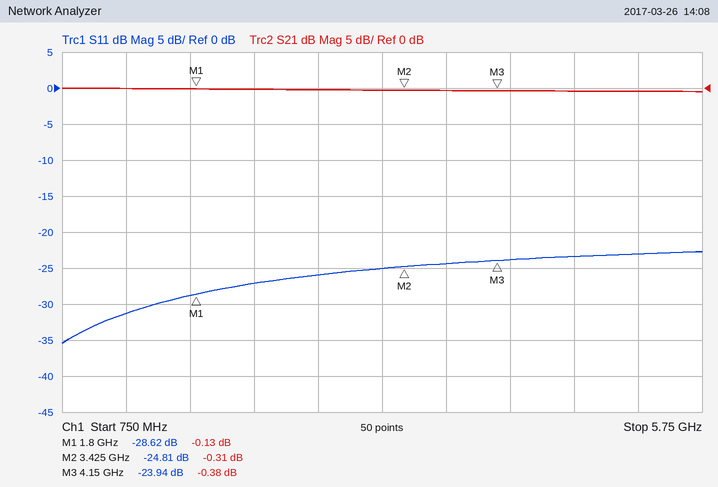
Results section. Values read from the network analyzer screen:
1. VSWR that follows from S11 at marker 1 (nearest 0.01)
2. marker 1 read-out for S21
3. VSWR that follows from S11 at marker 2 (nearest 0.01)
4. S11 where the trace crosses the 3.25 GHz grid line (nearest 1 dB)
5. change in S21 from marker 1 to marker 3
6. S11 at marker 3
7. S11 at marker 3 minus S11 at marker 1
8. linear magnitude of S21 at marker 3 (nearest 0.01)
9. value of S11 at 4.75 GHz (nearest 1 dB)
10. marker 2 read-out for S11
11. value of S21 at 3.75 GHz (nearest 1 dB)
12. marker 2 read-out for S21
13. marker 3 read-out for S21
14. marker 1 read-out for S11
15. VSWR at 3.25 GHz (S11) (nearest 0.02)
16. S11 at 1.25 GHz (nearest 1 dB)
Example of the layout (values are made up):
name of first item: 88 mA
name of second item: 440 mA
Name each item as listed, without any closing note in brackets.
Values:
VSWR that follows from S11 at marker 1: 1.08
marker 1 read-out for S21: -0.13 dB
VSWR that follows from S11 at marker 2: 1.12
S11 where the trace crosses the 3.25 GHz grid line: -25 dB
change in S21 from marker 1 to marker 3: -0.25 dB
S11 at marker 3: -23.94 dB
S11 at marker 3 minus S11 at marker 1: 4.68 dB
linear magnitude of S21 at marker 3: 0.96
value of S11 at 4.75 GHz: -23 dB
marker 2 read-out for S11: -24.81 dB
value of S21 at 3.75 GHz: 0 dB
marker 2 read-out for S21: -0.31 dB
marker 3 read-out for S21: -0.38 dB
marker 1 read-out for S11: -28.62 dB
VSWR at 3.25 GHz (S11): 1.12
S11 at 1.25 GHz: -31 dB
